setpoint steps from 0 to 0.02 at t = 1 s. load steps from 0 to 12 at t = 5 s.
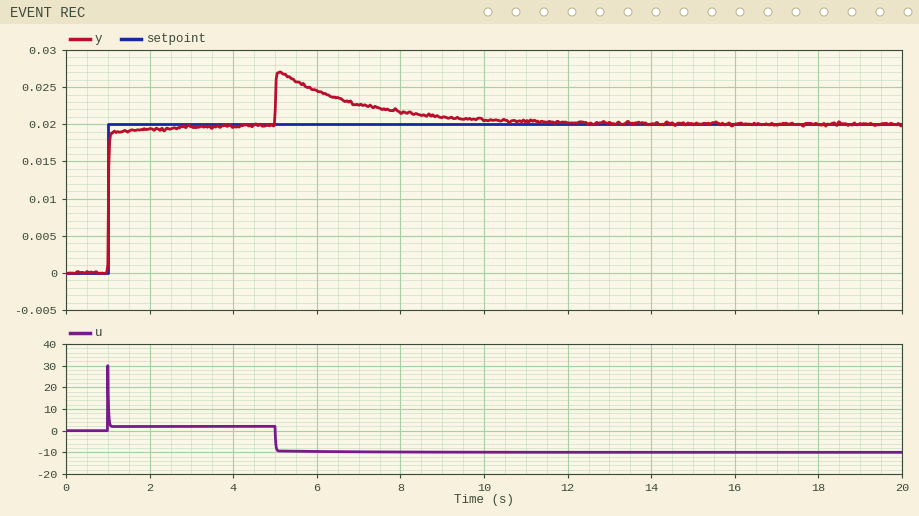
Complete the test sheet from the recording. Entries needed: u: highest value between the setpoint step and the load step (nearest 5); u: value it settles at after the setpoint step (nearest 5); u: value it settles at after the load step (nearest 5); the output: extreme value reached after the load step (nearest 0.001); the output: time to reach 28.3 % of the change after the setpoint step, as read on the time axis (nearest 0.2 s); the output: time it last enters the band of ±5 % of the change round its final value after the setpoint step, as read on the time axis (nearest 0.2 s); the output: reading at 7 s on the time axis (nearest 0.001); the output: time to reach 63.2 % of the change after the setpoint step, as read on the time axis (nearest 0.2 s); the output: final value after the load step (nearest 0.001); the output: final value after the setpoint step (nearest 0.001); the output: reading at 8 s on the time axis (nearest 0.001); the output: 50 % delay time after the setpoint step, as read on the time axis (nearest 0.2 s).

30
0
-10
0.027
1.0 s
1.2 s
0.023
1.0 s
0.020
0.020
0.022
1.0 s
